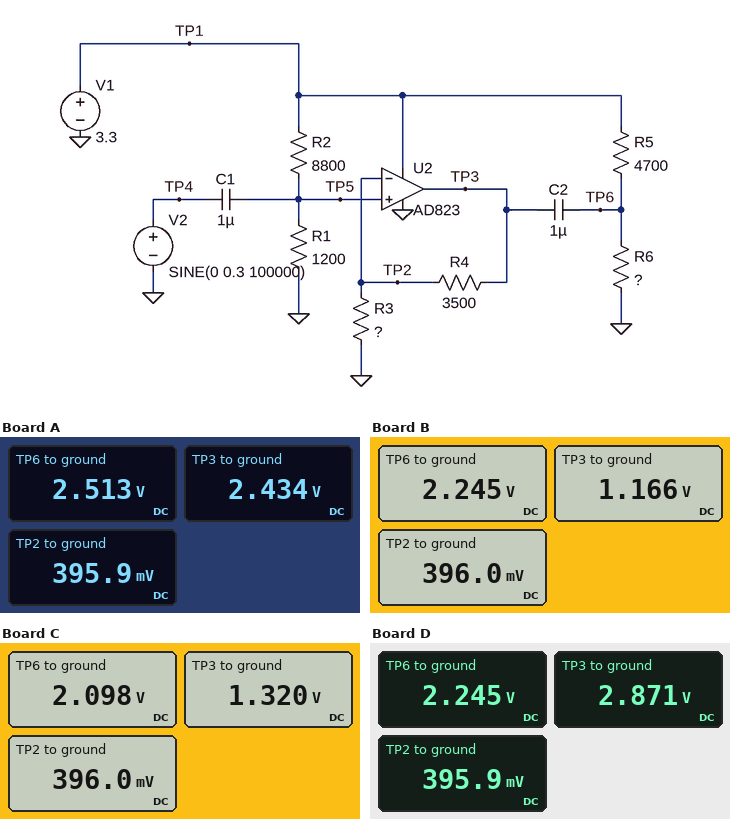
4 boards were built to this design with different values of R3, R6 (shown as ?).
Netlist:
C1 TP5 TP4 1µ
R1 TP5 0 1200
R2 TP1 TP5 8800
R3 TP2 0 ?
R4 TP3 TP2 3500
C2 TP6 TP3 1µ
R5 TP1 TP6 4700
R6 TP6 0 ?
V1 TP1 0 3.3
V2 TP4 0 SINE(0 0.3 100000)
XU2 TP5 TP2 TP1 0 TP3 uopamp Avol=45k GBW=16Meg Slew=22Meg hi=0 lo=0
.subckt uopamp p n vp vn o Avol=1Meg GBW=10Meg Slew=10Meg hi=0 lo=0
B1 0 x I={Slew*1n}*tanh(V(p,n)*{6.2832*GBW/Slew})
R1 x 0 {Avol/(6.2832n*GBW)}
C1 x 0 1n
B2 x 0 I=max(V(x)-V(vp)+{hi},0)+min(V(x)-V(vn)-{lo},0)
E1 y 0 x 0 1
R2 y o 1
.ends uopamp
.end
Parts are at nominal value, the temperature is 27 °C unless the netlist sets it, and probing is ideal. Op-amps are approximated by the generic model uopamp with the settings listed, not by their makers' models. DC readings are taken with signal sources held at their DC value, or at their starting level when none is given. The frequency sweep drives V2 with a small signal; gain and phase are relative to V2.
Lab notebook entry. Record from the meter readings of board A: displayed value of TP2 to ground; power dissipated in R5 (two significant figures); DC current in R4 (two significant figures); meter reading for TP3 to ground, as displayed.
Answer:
395.9 mV
130 µW
580 µA
2.434 V
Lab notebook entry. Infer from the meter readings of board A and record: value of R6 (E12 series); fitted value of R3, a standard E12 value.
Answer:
15 kΩ
680 Ω
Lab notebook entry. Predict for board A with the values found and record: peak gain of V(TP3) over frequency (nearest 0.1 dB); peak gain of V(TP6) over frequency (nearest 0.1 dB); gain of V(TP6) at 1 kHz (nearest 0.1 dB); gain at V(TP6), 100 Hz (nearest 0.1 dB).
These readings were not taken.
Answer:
15.8 dB
15.8 dB
15.7 dB
9.8 dB
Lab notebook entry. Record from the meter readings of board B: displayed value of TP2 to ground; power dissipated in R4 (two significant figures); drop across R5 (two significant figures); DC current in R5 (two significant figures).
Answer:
396.0 mV
170 µW
1.1 V
220 µA
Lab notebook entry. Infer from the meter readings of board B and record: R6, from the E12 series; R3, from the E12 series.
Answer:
10 kΩ
1.8 kΩ
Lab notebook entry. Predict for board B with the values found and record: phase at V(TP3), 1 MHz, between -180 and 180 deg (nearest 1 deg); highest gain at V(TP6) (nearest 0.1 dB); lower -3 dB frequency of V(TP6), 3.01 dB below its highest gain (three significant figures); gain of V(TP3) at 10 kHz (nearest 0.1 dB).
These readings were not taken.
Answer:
-10 deg
9.4 dB
165 Hz
9.4 dB
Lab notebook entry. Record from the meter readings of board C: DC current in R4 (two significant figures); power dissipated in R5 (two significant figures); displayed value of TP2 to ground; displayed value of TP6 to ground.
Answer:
260 µA
310 µW
396.0 mV
2.098 V
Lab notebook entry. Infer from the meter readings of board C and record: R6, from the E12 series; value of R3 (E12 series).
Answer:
8.2 kΩ
1.5 kΩ
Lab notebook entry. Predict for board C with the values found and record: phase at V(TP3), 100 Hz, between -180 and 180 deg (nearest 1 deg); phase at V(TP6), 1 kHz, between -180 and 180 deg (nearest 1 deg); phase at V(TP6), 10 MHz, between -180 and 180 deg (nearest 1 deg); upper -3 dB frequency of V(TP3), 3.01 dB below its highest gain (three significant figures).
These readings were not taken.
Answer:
56 deg
12 deg
-64 deg
4.80 MHz
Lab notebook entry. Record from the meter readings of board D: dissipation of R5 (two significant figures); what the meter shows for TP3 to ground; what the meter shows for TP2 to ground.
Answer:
240 µW
2.871 V
395.9 mV
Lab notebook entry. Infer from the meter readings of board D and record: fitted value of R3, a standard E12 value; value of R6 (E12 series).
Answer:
560 Ω
10 kΩ
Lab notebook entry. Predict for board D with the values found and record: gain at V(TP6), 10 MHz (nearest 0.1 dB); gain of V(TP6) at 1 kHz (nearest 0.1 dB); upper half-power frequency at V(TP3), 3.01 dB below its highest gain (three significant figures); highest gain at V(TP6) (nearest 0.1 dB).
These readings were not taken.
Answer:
3.9 dB
17.1 dB
2.21 MHz
17.2 dB
